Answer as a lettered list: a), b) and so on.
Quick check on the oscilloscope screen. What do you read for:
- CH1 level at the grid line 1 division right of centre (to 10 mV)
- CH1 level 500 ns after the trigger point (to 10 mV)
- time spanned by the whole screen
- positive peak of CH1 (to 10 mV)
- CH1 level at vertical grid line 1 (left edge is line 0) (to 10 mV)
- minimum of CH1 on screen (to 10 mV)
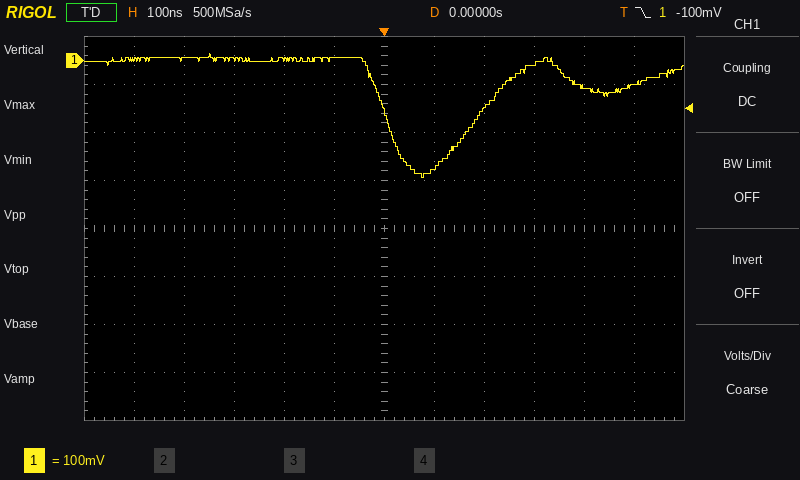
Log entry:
a) -220 mV
b) -50 mV
c) 1.2 µs
d) 10 mV
e) 0 mV
f) -240 mV
